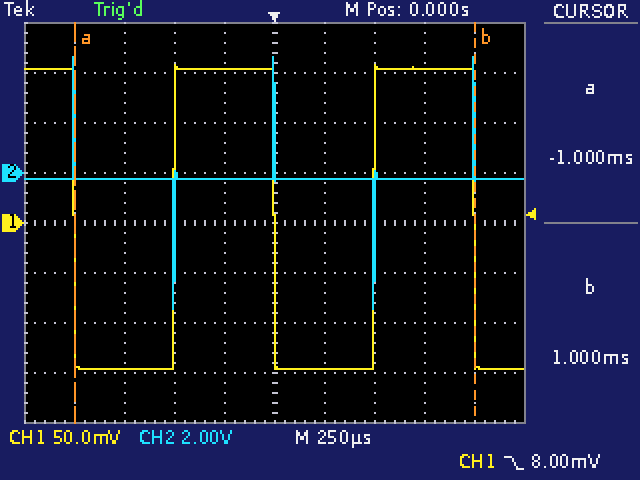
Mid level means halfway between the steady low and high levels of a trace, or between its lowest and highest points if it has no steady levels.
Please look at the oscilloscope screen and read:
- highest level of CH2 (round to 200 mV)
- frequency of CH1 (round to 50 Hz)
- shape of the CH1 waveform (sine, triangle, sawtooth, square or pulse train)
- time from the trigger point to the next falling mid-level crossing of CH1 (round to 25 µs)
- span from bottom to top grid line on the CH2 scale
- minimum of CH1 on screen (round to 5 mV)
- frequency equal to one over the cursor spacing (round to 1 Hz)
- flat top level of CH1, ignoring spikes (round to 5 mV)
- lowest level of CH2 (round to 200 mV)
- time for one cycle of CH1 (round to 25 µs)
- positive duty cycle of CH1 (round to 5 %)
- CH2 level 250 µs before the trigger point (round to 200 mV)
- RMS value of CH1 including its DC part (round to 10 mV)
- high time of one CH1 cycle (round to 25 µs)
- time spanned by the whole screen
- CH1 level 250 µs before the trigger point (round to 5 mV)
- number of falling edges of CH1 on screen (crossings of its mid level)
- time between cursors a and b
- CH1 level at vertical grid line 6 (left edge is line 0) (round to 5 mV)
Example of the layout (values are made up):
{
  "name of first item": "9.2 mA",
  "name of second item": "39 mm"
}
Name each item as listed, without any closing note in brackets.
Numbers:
{
  "highest level of CH2": "4.6 V",
  "frequency of CH1": "1.00 kHz",
  "shape of the CH1 waveform": "square",
  "time from the trigger point to the next falling mid-level crossing of CH1": "1.000 ms",
  "span from bottom to top grid line on the CH2 scale": "16 V",
  "minimum of CH1 on screen": "-145 mV",
  "frequency equal to one over the cursor spacing": "500 Hz",
  "flat top level of CH1, ignoring spikes": "155 mV",
  "lowest level of CH2": "-5.4 V",
  "time for one cycle of CH1": "1.000 ms",
  "positive duty cycle of CH1": "50 %",
  "CH2 level 250 µs before the trigger point": "-200 mV",
  "RMS value of CH1 including its DC part": "150 mV",
  "high time of one CH1 cycle": "500 µs",
  "time spanned by the whole screen": "2.5 ms",
  "CH1 level 250 µs before the trigger point": "155 mV",
  "number of falling edges of CH1 on screen": "3",
  "time between cursors a and b": "2.000 ms",
  "CH1 level at vertical grid line 6 (left edge is line 0)": "-145 mV"
}
